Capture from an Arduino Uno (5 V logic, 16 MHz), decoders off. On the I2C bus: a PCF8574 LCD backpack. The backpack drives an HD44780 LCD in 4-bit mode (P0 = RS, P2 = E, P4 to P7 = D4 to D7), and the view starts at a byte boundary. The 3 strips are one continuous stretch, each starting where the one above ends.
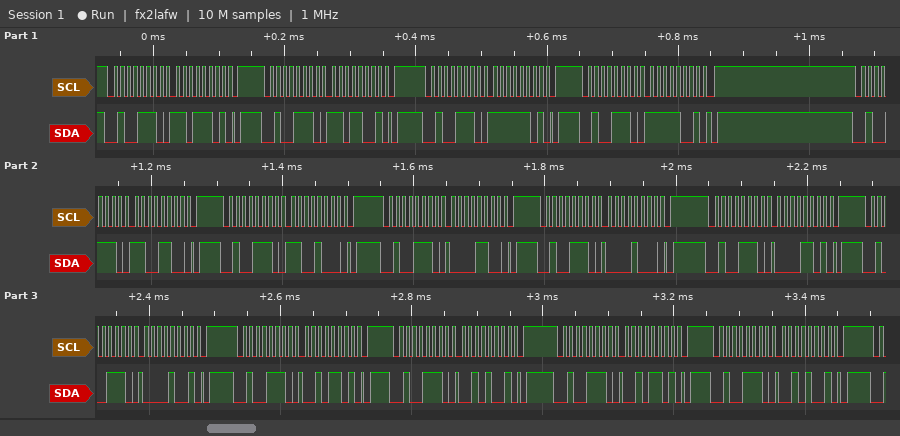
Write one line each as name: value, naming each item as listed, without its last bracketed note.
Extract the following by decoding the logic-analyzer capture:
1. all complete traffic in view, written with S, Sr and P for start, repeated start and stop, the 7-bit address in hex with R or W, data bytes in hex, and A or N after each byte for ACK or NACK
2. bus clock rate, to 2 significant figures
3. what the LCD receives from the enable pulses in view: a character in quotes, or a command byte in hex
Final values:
all complete traffic in view, written with S, Sr and P for start, repeated start and stop, the 7-bit address in hex with R or W, data bytes in hex, and A or N after each byte for ACK or NACK: S 27W A DD A P S 27W A D9 A P S 27W A FD A P S 27W A F9 A P S 27W A CC A P S 27W A C8 A P S 27W A 0C A P S 27W A 08 A P S 27W A 0D A P S 27W A 09 A P S 27W A 2D A P S 27W A 29 A P S 27W A 2D A P S 27W A 29 A P
bus clock rate, to 2 significant figures: 100 kHz
what the LCD receives from the enable pulses in view: a character in quotes, or a command byte in hex: data 0xDF 0xC0 data 0x02
